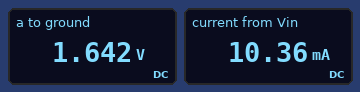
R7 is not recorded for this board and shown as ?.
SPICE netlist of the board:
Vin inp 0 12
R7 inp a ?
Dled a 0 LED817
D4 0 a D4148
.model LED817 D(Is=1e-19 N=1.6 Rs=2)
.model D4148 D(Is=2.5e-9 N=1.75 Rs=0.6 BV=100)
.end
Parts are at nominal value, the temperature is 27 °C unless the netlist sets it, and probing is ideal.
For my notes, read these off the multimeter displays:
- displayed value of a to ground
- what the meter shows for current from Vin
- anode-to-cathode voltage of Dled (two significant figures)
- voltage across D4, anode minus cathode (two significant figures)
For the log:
1.642 V
10.36 mA
1.6 V
-1.6 V
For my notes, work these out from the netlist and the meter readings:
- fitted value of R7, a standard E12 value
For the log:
1 kΩ
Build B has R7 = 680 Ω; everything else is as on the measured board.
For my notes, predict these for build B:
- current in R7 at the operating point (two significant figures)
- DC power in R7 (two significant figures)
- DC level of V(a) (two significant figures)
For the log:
15 mA
160 mW
1.7 V
